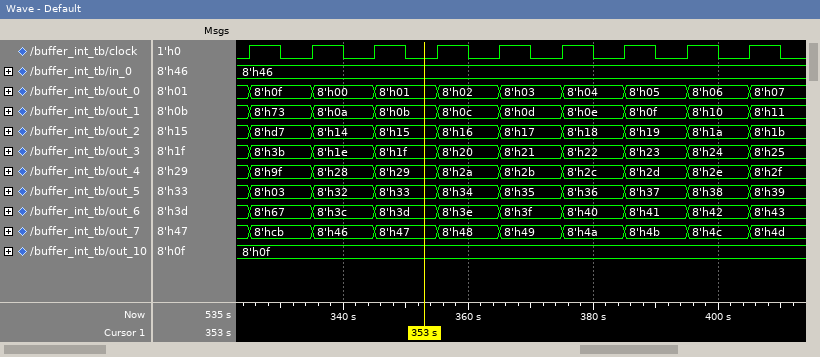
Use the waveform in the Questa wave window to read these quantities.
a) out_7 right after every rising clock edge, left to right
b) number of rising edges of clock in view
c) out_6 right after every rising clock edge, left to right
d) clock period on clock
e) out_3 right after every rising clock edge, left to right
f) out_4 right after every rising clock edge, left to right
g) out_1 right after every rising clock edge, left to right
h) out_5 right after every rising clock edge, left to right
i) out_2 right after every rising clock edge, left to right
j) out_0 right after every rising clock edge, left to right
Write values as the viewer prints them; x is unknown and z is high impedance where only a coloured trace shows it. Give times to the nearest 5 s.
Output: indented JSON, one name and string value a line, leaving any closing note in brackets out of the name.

{
  "out_7 right after every rising clock edge, left to right": "8'hcb, 8'h46, 8'h47, 8'h48, 8'h49, 8'h4a, 8'h4b, 8'h4c, 8'h4d",
  "number of rising edges of clock in view": "9",
  "out_6 right after every rising clock edge, left to right": "8'h67, 8'h3c, 8'h3d, 8'h3e, 8'h3f, 8'h40, 8'h41, 8'h42, 8'h43",
  "clock period on clock": "10 s",
  "out_3 right after every rising clock edge, left to right": "8'h3b, 8'h1e, 8'h1f, 8'h20, 8'h21, 8'h22, 8'h23, 8'h24, 8'h25",
  "out_4 right after every rising clock edge, left to right": "8'h9f, 8'h28, 8'h29, 8'h2a, 8'h2b, 8'h2c, 8'h2d, 8'h2e, 8'h2f",
  "out_1 right after every rising clock edge, left to right": "8'h73, 8'h0a, 8'h0b, 8'h0c, 8'h0d, 8'h0e, 8'h0f, 8'h10, 8'h11",
  "out_5 right after every rising clock edge, left to right": "8'h03, 8'h32, 8'h33, 8'h34, 8'h35, 8'h36, 8'h37, 8'h38, 8'h39",
  "out_2 right after every rising clock edge, left to right": "8'hd7, 8'h14, 8'h15, 8'h16, 8'h17, 8'h18, 8'h19, 8'h1a, 8'h1b",
  "out_0 right after every rising clock edge, left to right": "8'h0f, 8'h00, 8'h01, 8'h02, 8'h03, 8'h04, 8'h05, 8'h06, 8'h07"
}
